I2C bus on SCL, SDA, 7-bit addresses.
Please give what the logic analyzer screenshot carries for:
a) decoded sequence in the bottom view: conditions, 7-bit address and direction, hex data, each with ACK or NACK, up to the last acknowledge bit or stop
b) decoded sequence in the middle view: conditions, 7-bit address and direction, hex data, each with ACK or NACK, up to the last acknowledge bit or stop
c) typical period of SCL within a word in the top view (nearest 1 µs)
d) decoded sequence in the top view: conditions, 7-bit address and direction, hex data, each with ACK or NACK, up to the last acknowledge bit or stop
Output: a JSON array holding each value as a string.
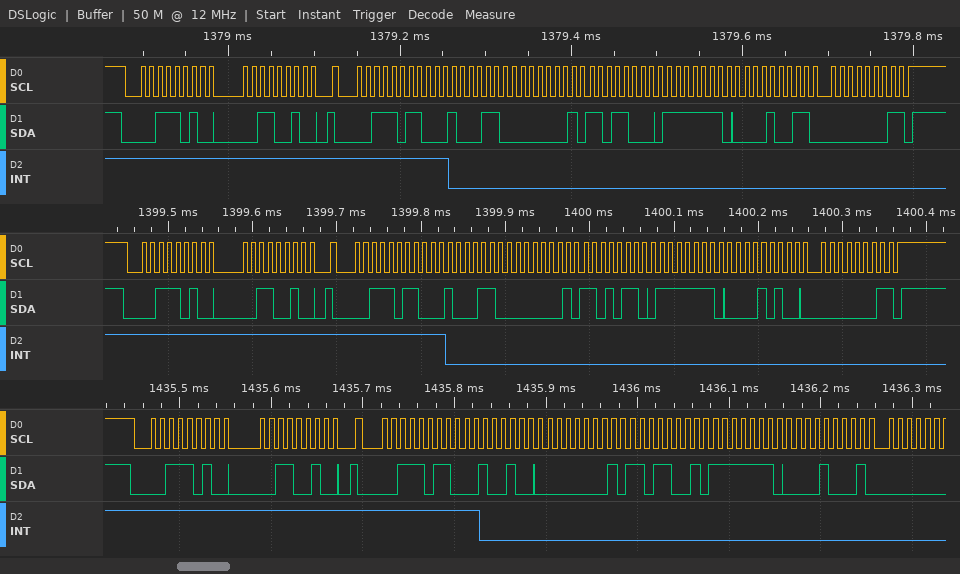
["start, address 1D write ACK, 32 ACK, repeated start, address 1D read ACK, 24 ACK, 01 ACK, D9 ACK, FE ACK, 11 ACK", "start, address 1D write ACK, 32 ACK, repeated start, address 1D read ACK, 23 ACK, 01 ACK, D6 ACK, FE ACK, 14 ACK, 01 NACK, stop", "10 µs", "start, address 1D write ACK, 32 ACK, repeated start, address 1D read ACK, 23 ACK, 01 ACK, D8 ACK, FE ACK, 13 ACK, 01 NACK, stop"]
